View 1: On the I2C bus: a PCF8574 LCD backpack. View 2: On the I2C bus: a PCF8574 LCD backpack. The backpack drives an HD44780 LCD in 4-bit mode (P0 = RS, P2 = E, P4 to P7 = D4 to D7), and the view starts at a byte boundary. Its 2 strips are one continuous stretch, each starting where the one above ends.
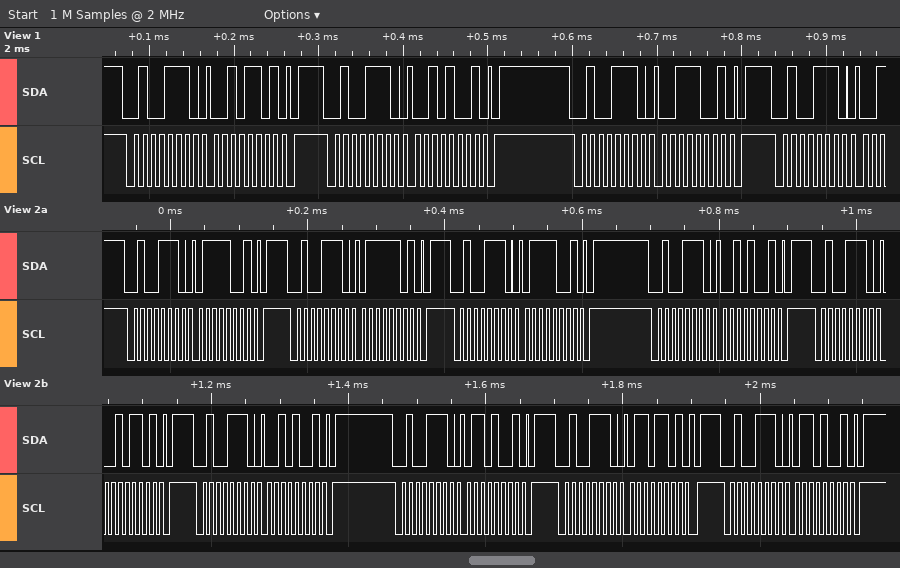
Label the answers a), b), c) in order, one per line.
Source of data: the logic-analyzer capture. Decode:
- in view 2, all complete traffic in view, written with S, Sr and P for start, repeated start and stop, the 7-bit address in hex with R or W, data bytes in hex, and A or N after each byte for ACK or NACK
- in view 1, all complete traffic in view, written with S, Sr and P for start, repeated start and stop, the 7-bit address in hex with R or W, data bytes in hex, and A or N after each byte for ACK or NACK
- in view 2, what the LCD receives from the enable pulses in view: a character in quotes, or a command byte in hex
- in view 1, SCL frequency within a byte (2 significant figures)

a) S 27W A 79 A P S 27W A 7D A P S 27W A 79 A P S 27W A 29 A P S 27W A 2D A P S 27W A 29 A P S 27W A 69 A P S 27W A 6D A P S 27W A 69 A P
b) S 27W A 2D A P S 27W A 29 A P S 27W A 39 A P S 27W A
c) 'r'
d) 100 kHz
